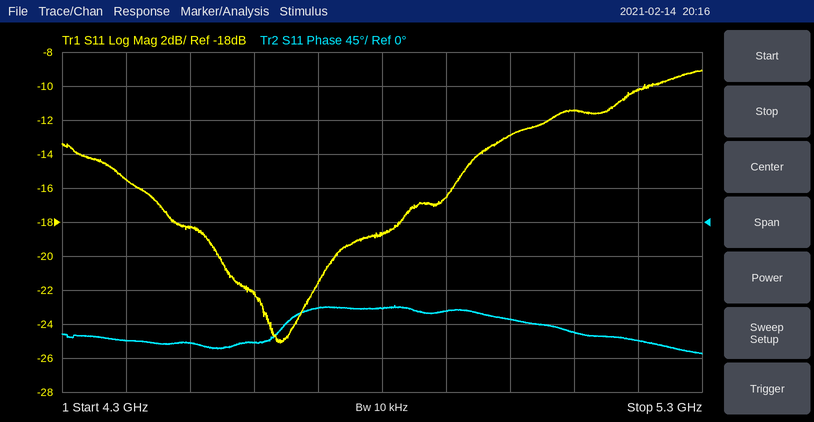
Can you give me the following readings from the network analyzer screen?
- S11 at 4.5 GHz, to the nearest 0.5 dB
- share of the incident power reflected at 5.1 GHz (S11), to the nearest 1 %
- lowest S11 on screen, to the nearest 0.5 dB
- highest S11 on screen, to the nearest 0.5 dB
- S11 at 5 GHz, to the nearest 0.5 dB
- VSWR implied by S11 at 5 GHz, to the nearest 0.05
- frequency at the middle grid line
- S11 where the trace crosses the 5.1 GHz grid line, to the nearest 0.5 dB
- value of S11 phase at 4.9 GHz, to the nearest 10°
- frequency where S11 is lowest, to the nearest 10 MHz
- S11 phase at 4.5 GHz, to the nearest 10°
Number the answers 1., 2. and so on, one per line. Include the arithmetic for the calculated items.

1. -18.5 dB
2. 10^(-11.5/10) ≈ 7 %
3. -25.0 dB
4. -9.0 dB
5. -13.0 dB
6. |Γ| = 10^(-13/20) = 0.2239; VSWR = (1 + 0.2239)/(1 − 0.2239) ≈ 1.58, so 1.60 to the nearest 0.05
7. 4.8 GHz
8. -11.5 dB
9. -120°
10. 4.64 GHz
11. -160°
